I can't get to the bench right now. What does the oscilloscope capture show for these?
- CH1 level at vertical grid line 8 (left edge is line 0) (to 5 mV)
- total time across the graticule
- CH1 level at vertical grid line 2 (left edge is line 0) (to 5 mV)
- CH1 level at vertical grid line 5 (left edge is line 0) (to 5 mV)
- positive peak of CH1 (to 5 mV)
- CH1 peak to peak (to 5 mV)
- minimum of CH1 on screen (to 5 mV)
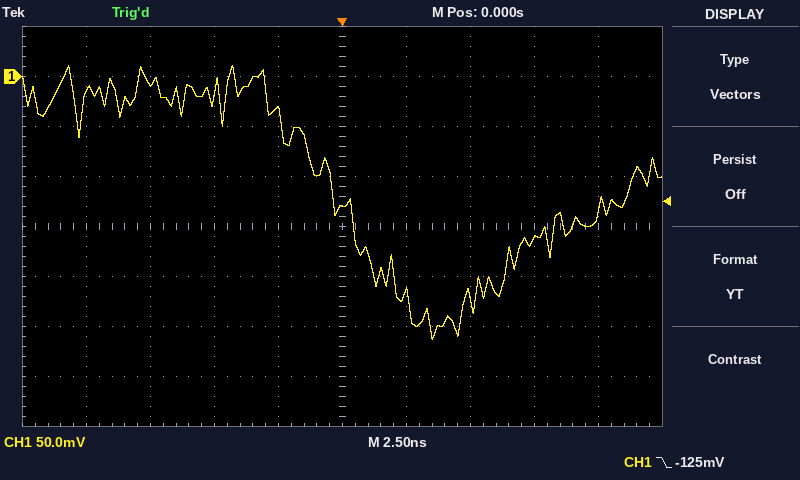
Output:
-165 mV
25 ns
-5 mV
-130 mV
10 mV
275 mV
-265 mV
